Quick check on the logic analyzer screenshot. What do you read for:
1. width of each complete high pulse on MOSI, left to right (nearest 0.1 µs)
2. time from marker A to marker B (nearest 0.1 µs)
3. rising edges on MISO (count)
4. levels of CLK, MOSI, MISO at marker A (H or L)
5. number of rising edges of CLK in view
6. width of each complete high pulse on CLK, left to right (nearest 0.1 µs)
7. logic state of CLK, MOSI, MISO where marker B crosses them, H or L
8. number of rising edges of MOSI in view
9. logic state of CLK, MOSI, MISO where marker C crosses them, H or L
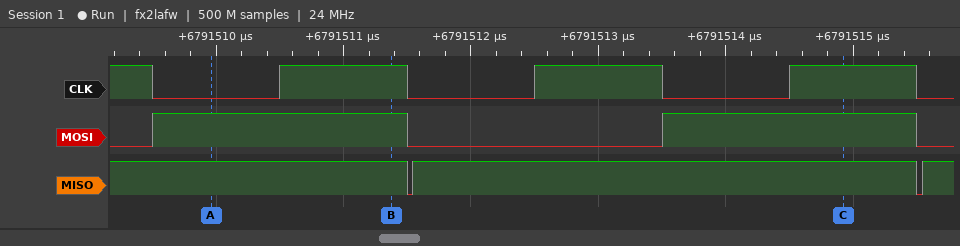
2 µs, 2 µs
1.4 µs
2
CLK=L, MOSI=H, MISO=H
3
1 µs, 1 µs, 1 µs
CLK=H, MOSI=H, MISO=H
2
CLK=H, MOSI=H, MISO=H
